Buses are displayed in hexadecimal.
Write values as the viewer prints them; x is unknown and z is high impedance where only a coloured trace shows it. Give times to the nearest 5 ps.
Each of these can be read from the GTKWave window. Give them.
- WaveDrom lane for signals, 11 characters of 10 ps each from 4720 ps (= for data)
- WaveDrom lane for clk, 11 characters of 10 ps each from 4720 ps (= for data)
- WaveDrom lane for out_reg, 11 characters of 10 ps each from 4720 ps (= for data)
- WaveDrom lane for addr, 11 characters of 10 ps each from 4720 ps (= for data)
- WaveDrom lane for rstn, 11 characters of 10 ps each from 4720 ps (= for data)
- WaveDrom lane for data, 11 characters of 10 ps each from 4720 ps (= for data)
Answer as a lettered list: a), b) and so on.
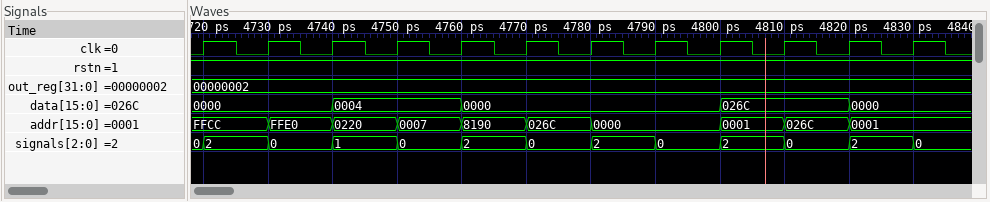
a) {name: 'signals', wave: '===========', data: '2 0 1 0 2 0 2 0 2 0 2'}
b) {name: 'clk', wave: 'p..........'}
c) {name: 'out_reg', wave: '=..........', data: '00000002'}
d) {name: 'addr', wave: '=======.===', data: 'FFCC FFE0 0220 0007 8190 026C 0000 0001 026C 0001'}
e) {name: 'rstn', wave: '1..........'}
f) {name: 'data', wave: '=.=.=...=.=', data: '0000 0004 0000 026C 0000'}
